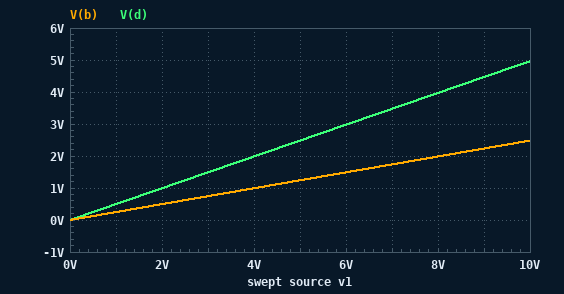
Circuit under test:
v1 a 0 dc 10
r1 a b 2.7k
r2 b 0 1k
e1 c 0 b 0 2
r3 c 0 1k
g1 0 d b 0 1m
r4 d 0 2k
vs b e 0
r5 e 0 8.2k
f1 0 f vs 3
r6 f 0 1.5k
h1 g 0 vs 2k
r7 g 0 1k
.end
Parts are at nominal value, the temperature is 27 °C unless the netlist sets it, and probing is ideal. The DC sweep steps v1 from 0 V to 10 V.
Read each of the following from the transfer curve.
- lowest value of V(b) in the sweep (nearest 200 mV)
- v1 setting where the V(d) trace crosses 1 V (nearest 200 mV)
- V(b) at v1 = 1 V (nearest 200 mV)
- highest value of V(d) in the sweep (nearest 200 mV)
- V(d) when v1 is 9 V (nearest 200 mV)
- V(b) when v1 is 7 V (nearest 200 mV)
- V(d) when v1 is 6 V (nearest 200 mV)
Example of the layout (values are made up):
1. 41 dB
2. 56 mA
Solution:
1. 0 V
2. 2.0 V
3. 200 mV
4. 5.0 V
5. 4.4 V
6. 1.8 V
7. 3.0 V
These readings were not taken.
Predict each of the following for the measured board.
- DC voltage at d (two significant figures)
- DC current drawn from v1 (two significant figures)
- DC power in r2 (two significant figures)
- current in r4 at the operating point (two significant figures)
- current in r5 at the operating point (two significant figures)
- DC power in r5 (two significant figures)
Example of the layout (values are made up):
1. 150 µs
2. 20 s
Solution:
1. 5.0 V
2. 2.8 mA
3. 6.2 mW
4. 2.5 mA
5. 300 µA
6. 750 µW
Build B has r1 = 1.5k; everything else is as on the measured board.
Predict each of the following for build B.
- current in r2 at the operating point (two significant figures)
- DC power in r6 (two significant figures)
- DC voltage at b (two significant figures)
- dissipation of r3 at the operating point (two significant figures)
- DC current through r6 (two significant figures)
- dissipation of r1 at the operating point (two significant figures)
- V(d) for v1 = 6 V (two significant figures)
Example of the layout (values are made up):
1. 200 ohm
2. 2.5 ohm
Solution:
1. 3.7 mA
2. 2.8 mW
3. 3.7 V
4. 56 mW
5. 1.4 mA
6. 26 mW
7. 4.5 V
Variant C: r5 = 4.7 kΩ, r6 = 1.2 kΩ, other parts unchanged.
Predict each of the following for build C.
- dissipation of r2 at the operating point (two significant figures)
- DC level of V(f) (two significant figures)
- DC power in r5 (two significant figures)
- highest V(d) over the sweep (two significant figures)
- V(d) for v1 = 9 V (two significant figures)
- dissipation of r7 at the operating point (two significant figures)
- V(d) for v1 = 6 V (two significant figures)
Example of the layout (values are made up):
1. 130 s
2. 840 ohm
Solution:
1. 5.5 mW
2. 1.8 V
3. 1.2 mW
4. 4.7 V
5. 4.2 V
6. 990 µW
7. 2.8 V
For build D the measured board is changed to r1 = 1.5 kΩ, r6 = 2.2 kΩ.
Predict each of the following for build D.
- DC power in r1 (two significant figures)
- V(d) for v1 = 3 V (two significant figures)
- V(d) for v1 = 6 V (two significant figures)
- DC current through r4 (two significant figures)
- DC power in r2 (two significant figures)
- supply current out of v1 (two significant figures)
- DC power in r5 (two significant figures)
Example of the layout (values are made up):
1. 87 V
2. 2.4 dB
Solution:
1. 26 mW
2. 2.2 V
3. 4.5 V
4. 3.7 mA
5. 14 mW
6. 4.2 mA
7. 1.7 mW
